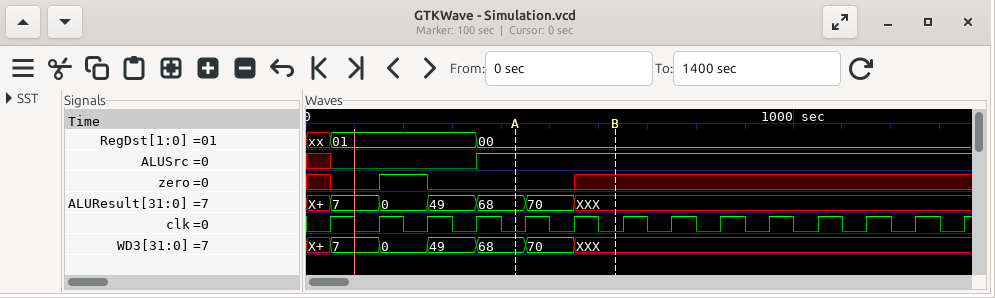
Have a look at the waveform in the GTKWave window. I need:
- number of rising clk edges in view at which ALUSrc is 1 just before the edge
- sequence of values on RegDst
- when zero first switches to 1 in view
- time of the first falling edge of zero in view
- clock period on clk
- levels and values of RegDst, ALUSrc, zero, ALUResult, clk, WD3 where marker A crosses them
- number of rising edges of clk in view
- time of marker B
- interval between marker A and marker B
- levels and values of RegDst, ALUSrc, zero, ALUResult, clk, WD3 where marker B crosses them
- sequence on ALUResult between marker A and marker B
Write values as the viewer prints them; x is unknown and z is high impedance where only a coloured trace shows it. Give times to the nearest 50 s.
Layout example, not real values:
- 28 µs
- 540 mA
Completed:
- 10
- xx, 01, 00
- 150 s
- 250 s
- 100 s
- RegDst=00, ALUSrc=1, zero=0, ALUResult=68, clk=0, WD3=68
- 14
- 650 s
- 200 s
- RegDst=00, ALUSrc=1, zero=x, ALUResult=XXX, clk=0, WD3=XXX
- 68, 70, XXX
